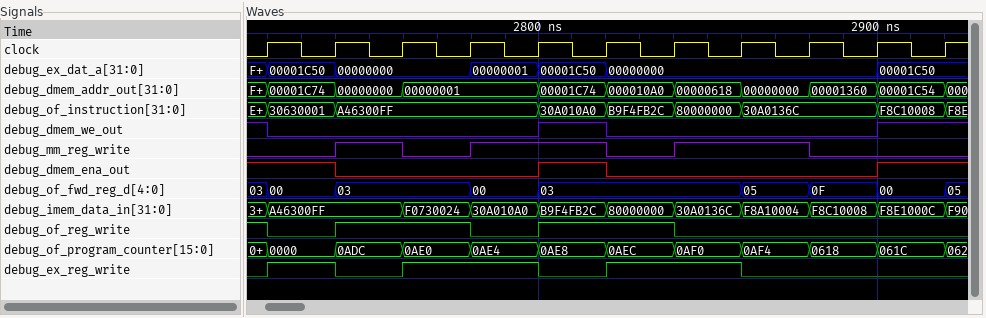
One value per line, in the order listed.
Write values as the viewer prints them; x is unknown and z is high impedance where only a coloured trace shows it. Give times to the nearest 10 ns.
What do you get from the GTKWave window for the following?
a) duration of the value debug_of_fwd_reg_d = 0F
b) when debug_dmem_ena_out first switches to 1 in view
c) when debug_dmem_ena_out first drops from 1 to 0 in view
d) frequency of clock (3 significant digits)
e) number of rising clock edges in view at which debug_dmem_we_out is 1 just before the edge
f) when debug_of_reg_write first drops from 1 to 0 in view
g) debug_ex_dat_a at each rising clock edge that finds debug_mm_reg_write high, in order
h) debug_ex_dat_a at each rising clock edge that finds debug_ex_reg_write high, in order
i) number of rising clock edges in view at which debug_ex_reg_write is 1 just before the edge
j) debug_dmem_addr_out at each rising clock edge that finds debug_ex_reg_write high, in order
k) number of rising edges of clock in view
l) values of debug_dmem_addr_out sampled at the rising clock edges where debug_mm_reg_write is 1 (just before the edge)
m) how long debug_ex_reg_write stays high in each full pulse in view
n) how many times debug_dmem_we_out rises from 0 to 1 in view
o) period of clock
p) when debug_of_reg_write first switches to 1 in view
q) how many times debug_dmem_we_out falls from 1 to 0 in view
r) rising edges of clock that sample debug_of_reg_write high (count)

20 ns
2800 ns
2740 ns
50.0 MHz
3
2720 ns
00000000, 00000001, 00001C50, 00000000, 00000000
00001C50, 00000000, 00000001, 00000000, 00000000
5
00001C74, 00000001, 00000001, 000010A0, 00000618
11
00000000, 00000001, 00001C74, 00000618, 00000000
20 ns, 40 ns, 40 ns
2
20 ns
2740 ns
2
5
